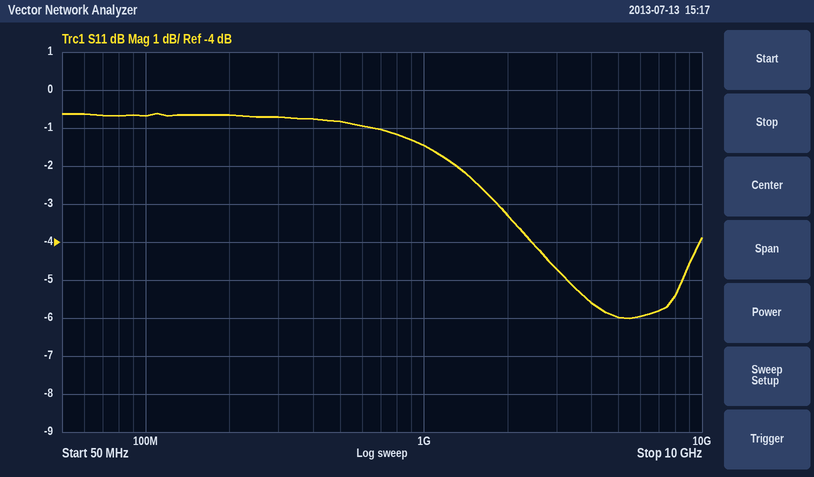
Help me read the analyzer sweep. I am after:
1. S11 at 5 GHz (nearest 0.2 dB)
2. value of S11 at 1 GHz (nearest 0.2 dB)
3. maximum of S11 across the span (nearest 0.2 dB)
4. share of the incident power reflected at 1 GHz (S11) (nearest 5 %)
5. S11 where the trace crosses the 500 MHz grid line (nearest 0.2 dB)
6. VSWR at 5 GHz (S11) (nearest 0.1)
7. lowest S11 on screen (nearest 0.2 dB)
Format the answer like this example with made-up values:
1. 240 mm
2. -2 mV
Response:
1. -6.0 dB
2. -1.4 dB
3. -0.6 dB
4. 70 %
5. -0.8 dB
6. 3.0
7. -6.0 dB
